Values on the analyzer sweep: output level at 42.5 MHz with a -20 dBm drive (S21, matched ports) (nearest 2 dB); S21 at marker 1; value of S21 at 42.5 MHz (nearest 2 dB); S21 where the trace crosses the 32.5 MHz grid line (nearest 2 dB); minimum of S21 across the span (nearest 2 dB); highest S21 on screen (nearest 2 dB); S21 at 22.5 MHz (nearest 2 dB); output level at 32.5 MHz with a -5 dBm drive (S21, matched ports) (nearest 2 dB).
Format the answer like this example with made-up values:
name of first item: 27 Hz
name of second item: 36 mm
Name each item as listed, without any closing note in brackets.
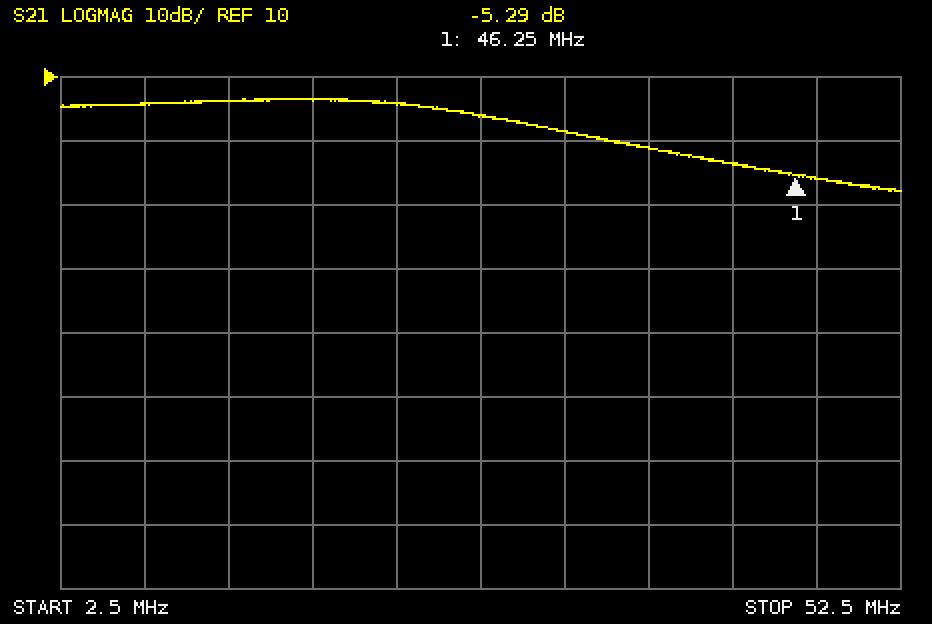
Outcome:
output level at 42.5 MHz with a -20 dBm drive (S21, matched ports): -24 dBm
S21 at marker 1: -5.29 dB
value of S21 at 42.5 MHz: -4 dB
S21 where the trace crosses the 32.5 MHz grid line: 2 dB
minimum of S21 across the span: -8 dB
highest S21 on screen: 6 dB
S21 at 22.5 MHz: 6 dB
output level at 32.5 MHz with a -5 dBm drive (S21, matched ports): -4 dBm
